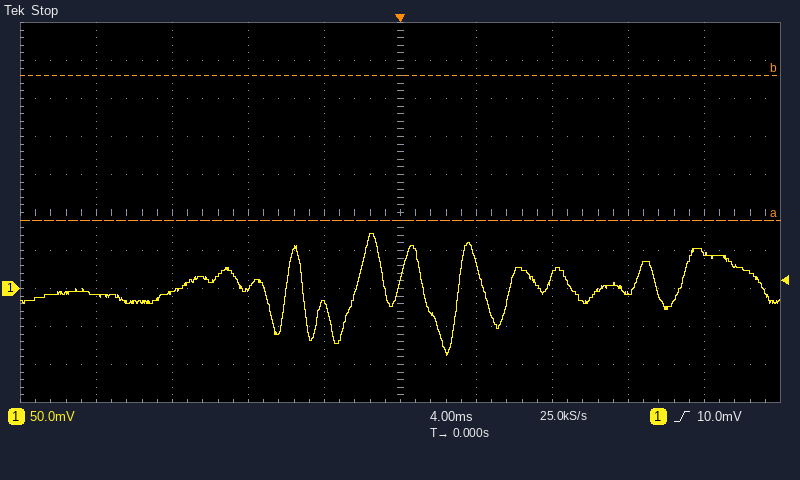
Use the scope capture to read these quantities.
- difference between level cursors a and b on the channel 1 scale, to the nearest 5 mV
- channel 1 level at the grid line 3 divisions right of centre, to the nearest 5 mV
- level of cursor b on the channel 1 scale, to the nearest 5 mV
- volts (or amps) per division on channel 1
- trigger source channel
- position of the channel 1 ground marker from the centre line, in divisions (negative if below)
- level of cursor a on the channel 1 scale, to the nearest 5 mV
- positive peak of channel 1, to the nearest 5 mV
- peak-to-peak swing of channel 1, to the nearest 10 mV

190 mV
-5 mV
280 mV
50 mV
channel 1
-2.0 div
90 mV
70 mV
160 mV
